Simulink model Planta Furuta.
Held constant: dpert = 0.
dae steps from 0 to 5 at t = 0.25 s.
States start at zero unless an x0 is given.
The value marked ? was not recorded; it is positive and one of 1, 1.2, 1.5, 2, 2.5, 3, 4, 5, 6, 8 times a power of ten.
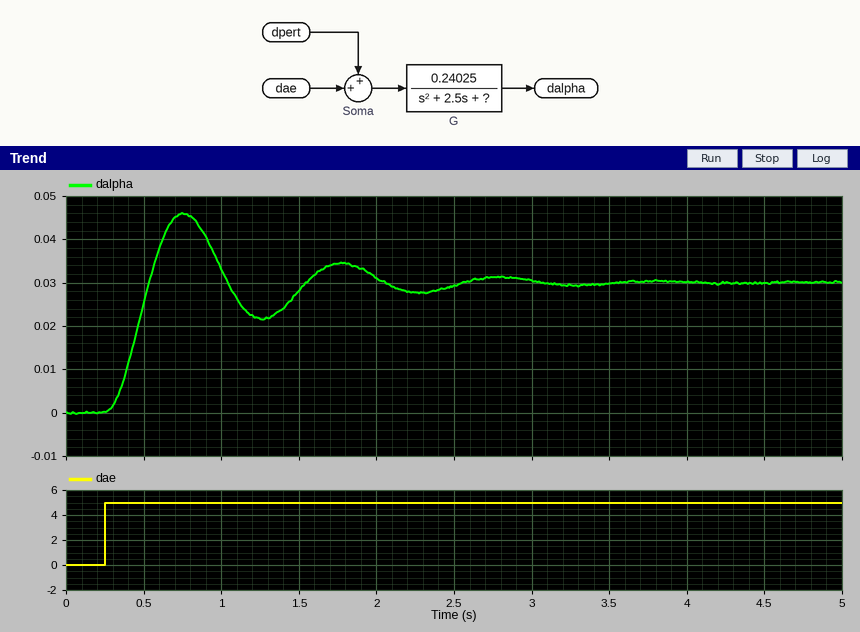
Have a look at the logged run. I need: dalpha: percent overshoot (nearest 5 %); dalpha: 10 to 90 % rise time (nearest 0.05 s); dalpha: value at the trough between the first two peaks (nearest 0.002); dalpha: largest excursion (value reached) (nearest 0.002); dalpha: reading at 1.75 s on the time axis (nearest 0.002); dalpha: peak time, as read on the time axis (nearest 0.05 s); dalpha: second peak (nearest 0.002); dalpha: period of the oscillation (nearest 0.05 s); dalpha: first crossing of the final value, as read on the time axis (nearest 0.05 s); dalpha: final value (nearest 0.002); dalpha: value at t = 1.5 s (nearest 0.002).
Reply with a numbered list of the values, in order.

1. 55 %
2. 0.20 s
3. 0.022
4. 0.046
5. 0.034
6. 0.75 s
7. 0.034
8. 1.00 s
9. 0.55 s
10. 0.030
11. 0.028
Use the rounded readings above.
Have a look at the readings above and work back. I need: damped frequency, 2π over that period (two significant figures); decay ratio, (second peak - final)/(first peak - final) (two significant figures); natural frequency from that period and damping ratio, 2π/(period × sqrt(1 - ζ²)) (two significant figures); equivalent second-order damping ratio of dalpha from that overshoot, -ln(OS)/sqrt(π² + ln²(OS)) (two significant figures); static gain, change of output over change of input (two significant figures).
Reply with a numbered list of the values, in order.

1. 6.3 rad/s
2. 0.25
3. 6.4 rad/s
4. 0.19
5. 0.0060
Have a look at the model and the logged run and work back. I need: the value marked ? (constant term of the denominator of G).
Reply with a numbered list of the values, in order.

1. 40
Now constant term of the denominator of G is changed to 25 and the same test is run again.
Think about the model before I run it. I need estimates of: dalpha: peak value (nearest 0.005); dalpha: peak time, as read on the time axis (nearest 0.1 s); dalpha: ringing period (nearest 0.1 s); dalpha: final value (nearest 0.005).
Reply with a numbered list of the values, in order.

1. 0.070
2. 0.9 s
3. 1.3 s
4. 0.050
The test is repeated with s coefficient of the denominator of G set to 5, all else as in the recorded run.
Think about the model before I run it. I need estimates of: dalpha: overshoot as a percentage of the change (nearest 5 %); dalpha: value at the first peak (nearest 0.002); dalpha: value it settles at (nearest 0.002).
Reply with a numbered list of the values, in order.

1. 25 %
2. 0.038
3. 0.030
